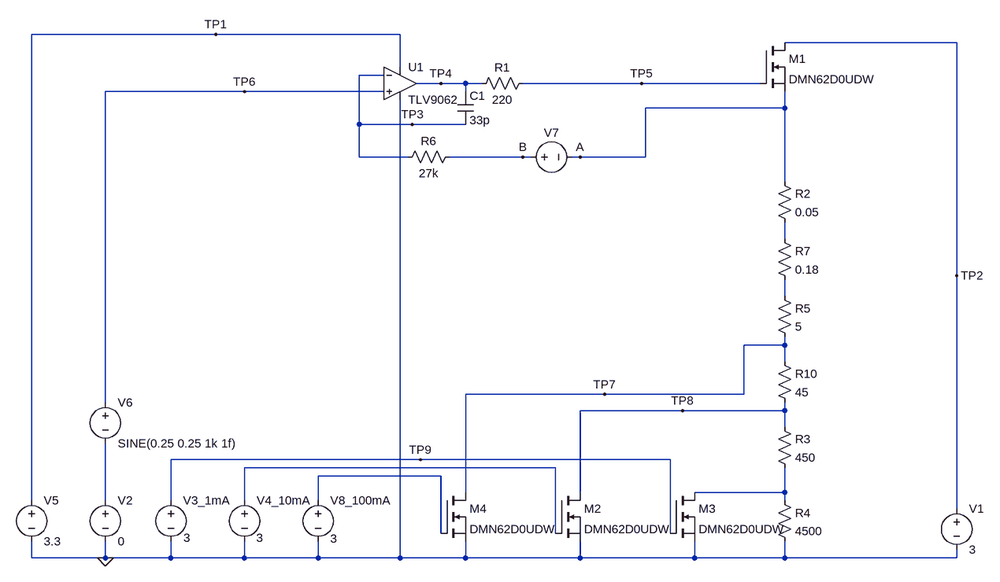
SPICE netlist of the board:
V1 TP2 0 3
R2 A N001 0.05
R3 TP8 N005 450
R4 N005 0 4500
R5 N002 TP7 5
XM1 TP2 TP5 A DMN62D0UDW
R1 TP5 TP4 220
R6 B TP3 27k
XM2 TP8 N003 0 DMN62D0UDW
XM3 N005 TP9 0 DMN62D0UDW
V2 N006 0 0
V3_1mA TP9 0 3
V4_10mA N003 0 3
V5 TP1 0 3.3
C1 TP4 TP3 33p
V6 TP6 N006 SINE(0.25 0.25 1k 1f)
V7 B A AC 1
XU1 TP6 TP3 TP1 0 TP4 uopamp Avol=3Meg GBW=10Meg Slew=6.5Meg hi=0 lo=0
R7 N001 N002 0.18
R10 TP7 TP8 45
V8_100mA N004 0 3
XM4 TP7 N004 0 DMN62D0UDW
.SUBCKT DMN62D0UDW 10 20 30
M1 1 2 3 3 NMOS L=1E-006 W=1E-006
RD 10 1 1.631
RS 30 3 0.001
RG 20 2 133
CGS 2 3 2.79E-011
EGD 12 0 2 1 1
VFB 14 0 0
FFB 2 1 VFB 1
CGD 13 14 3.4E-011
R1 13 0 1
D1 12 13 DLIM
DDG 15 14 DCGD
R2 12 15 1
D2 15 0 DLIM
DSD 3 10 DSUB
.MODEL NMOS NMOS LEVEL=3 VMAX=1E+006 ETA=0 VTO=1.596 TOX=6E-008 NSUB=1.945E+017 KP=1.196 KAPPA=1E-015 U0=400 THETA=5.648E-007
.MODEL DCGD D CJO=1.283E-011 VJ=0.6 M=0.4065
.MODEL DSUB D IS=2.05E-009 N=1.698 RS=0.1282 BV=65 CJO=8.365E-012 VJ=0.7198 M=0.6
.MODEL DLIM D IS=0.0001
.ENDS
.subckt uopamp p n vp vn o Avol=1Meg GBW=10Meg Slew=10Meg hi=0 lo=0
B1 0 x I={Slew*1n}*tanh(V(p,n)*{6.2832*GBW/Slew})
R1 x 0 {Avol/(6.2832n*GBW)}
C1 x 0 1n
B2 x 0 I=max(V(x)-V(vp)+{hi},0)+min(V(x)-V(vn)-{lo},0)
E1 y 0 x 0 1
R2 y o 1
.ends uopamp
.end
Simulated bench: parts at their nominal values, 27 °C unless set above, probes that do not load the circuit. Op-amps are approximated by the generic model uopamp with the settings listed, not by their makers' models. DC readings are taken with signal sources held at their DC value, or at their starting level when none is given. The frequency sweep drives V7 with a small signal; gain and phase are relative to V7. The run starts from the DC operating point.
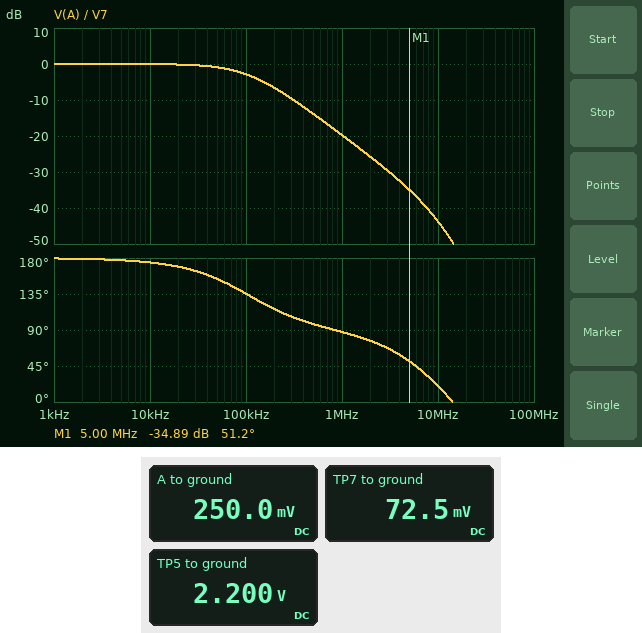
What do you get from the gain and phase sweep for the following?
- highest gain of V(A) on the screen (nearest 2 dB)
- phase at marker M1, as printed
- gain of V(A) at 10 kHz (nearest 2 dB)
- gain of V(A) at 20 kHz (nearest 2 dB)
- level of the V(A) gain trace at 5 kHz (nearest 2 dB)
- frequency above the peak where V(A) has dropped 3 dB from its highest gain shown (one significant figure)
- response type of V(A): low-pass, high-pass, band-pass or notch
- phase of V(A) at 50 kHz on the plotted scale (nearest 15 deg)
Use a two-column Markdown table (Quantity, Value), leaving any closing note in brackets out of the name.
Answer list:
| Quantity | Value |
|---|---|
| highest gain of V(A) on the screen | 0 dB |
| phase at marker M1, as printed | 51.2 deg |
| gain of V(A) at 10 kHz | 0 dB |
| gain of V(A) at 20 kHz | 0 dB |
| level of the V(A) gain trace at 5 kHz | 0 dB |
| frequency above the peak where V(A) has dropped 3 dB from its highest gain shown | 100 kHz |
| response type of V(A): low-pass, high-pass, band-pass or notch | low-pass |
| phase of V(A) at 50 kHz on the plotted scale | 150 deg |
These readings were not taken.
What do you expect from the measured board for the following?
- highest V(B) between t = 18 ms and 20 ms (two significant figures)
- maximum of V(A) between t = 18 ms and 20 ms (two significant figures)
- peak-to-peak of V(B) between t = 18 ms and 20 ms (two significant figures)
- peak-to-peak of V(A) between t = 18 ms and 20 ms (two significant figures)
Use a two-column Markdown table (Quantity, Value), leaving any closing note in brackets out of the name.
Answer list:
| Quantity | Value |
|---|---|
| highest V(B) between t = 18 ms and 20 ms | 500 mV |
| maximum of V(A) between t = 18 ms and 20 ms | 500 mV |
| peak-to-peak of V(B) between t = 18 ms and 20 ms | 500 mV |
| peak-to-peak of V(A) between t = 18 ms and 20 ms | 500 mV |
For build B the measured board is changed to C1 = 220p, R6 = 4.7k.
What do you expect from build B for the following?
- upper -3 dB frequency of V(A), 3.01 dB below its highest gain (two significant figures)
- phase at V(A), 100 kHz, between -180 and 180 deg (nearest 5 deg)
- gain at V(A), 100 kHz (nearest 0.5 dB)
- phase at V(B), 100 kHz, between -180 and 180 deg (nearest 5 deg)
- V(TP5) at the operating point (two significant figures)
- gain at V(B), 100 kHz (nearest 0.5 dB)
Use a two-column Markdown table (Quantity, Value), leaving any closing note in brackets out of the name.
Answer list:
| Quantity | Value |
|---|---|
| upper -3 dB frequency of V(A), 3.01 dB below its highest gain | 90 kHz |
| phase at V(A), 100 kHz, between -180 and 180 deg | 130 deg |
| gain at V(A), 100 kHz | -3.5 dB |
| phase at V(B), 100 kHz, between -180 and 180 deg | 40 deg |
| V(TP5) at the operating point | 2.2 V |
| gain at V(B), 100 kHz | -2.5 dB |
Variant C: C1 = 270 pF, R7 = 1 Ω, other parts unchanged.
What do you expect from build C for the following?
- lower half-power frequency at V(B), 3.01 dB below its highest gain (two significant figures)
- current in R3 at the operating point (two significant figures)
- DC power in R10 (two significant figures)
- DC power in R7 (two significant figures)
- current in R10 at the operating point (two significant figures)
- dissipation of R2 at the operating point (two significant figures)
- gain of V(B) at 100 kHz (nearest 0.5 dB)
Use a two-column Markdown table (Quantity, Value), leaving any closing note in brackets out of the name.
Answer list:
| Quantity | Value |
|---|---|
| lower half-power frequency at V(B), 3.01 dB below its highest gain | 13 kHz |
| current in R3 at the operating point | 6.8 µA |
| DC power in R10 | 86 µW |
| DC power in R7 | 930 µW |
| current in R10 at the operating point | 1.4 mA |
| dissipation of R2 at the operating point | 47 µW |
| gain of V(B) at 100 kHz | 0 dB |
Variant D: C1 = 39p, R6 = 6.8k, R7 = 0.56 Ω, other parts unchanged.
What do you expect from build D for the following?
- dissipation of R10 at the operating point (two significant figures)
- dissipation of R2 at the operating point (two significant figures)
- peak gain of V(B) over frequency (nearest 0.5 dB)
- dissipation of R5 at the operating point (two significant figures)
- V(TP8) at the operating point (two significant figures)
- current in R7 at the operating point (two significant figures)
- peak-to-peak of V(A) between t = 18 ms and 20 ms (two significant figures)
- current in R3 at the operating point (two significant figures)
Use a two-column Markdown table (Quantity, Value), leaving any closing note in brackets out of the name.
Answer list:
| Quantity | Value |
|---|---|
| dissipation of R10 at the operating point | 96 µW |
| dissipation of R2 at the operating point | 52 µW |
| peak gain of V(B) over frequency | 0.5 dB |
| dissipation of R5 at the operating point | 5.2 mW |
| V(TP8) at the operating point | 3.2 mV |
| current in R7 at the operating point | 32 mA |
| peak-to-peak of V(A) between t = 18 ms and 20 ms | 500 mV |
| current in R3 at the operating point | 7.2 µA |
